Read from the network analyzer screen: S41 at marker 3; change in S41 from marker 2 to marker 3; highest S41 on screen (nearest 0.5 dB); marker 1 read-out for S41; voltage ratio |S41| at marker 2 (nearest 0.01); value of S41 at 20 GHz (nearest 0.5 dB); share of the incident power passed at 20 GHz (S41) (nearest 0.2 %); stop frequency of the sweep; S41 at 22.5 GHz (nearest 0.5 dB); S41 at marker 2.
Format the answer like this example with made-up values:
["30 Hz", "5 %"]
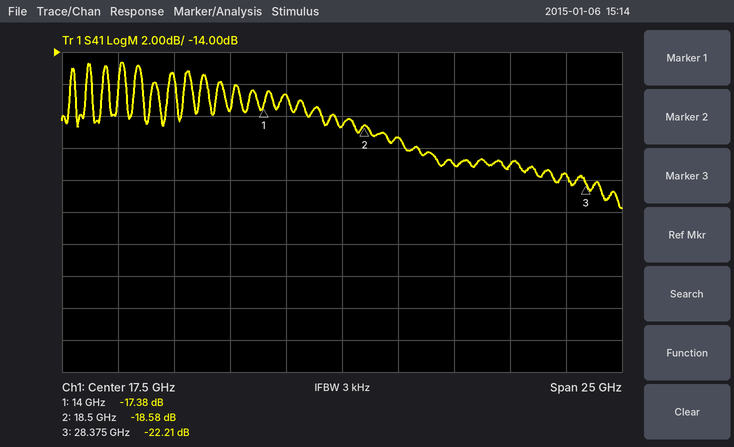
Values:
["-22.21 dB", "-3.63 dB", "-14.5 dB", "-17.38 dB", "0.12", "-19.5 dB", "1.2 %", "30 GHz", "-21.0 dB", "-18.58 dB"]
